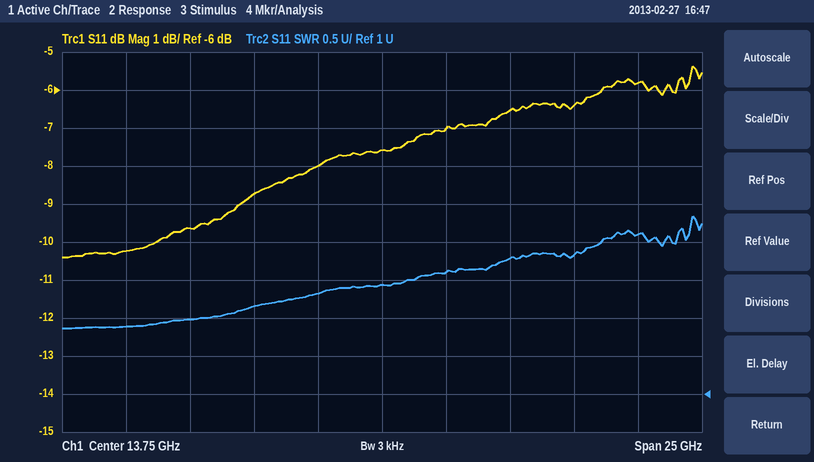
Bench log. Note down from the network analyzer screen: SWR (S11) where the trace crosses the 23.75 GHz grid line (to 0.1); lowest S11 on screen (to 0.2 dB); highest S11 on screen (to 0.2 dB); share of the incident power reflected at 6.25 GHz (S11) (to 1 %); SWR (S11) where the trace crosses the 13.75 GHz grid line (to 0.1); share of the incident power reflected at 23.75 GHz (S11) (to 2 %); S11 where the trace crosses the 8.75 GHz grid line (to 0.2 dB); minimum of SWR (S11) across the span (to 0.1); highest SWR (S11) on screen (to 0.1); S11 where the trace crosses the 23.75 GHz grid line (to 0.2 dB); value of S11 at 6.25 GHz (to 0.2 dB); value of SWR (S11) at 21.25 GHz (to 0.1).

3.1
-10.4 dB
-5.4 dB
11 %
2.4
26 %
-8.8 dB
1.9
3.3
-5.8 dB
-9.6 dB
2.8
